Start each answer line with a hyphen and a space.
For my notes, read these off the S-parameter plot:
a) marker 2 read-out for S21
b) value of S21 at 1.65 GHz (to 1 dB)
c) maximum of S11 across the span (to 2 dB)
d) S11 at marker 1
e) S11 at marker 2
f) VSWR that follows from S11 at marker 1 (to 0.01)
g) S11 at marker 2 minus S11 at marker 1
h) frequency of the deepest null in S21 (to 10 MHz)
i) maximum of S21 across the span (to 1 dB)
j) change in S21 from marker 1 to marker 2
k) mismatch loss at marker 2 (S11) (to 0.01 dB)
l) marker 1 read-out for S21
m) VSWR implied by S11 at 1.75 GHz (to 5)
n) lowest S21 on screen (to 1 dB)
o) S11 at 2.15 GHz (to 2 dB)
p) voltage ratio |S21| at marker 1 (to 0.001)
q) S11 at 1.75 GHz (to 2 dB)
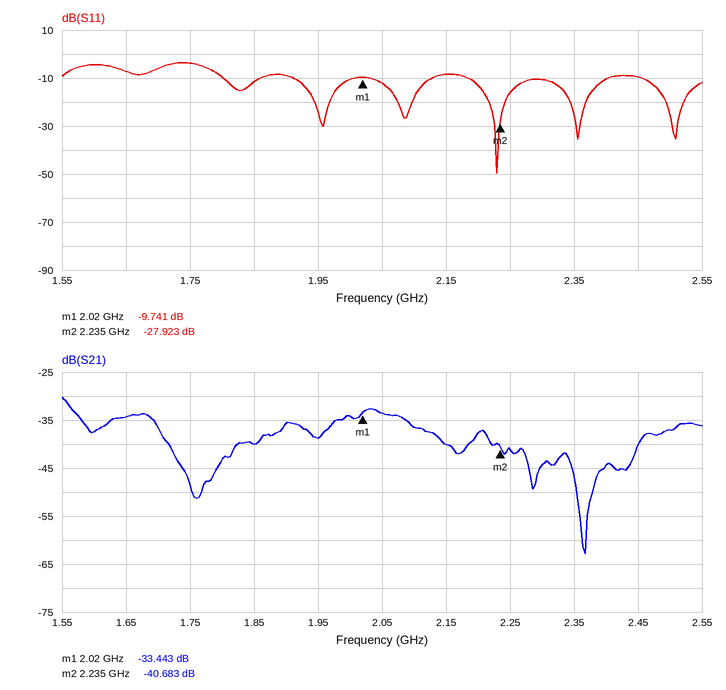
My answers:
- -40.683 dB
- -34 dB
- -4 dB
- -9.741 dB
- -27.923 dB
- 1.97
- -18.182 dB
- 2.37 GHz
- -30 dB
- -7.240 dB
- 0.01 dB
- -33.443 dB
- 5
- -63 dB
- -8 dB
- 0.021
- -4 dB
